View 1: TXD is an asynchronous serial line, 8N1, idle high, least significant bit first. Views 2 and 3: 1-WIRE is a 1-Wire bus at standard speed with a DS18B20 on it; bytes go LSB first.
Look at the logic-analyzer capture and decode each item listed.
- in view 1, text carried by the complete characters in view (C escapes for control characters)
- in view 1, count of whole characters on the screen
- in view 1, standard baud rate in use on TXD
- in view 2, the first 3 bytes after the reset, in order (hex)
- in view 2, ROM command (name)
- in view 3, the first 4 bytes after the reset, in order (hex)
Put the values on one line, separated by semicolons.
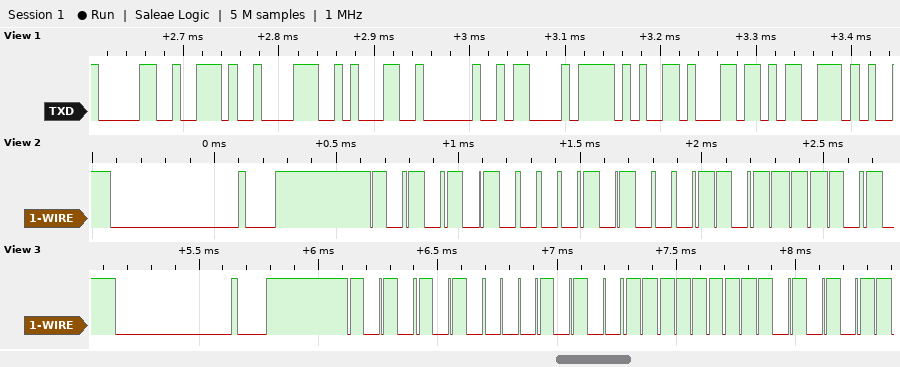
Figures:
"0.81 Cels"; 9; 115200 baud; 55 28 F6; Match ROM; 55 28 FF D5
